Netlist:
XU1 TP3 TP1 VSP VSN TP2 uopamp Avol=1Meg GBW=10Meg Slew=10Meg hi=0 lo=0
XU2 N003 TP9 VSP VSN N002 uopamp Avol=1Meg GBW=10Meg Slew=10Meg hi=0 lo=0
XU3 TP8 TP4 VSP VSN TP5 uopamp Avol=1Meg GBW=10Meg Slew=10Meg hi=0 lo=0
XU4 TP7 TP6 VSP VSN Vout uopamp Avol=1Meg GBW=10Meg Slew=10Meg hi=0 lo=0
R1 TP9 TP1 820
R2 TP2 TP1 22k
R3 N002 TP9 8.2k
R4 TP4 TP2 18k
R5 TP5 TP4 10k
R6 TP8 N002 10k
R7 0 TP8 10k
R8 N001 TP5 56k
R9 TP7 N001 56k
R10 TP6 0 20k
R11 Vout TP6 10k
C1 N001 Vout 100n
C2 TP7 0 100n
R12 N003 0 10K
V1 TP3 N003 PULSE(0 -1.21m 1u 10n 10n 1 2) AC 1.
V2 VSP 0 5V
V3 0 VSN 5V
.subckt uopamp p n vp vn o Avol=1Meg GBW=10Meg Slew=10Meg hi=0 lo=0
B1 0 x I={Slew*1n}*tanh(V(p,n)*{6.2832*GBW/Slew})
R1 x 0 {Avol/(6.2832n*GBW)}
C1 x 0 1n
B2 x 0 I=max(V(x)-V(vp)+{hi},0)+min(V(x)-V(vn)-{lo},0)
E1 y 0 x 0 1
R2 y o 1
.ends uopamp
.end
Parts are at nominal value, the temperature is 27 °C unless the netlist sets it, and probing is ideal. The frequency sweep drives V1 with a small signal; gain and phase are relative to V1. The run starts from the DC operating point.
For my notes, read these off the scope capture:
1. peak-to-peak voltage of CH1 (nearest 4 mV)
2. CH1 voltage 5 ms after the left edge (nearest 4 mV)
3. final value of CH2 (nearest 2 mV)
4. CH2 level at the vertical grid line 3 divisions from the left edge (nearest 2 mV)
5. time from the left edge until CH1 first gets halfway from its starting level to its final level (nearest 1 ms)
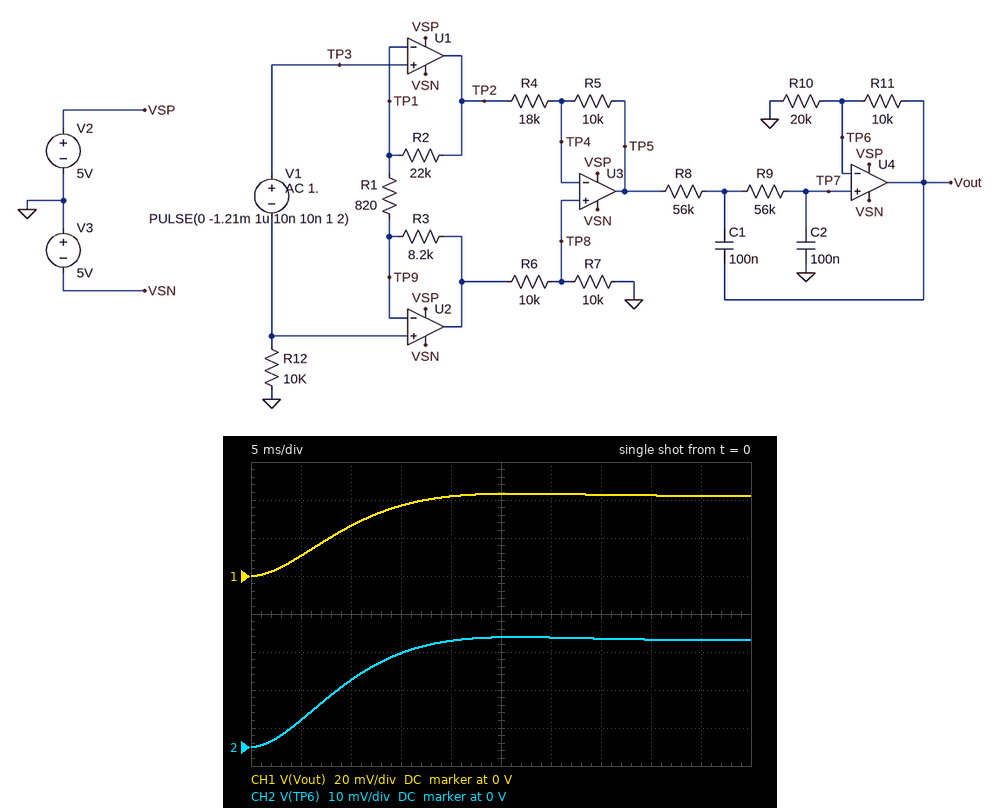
44 mV
12 mV
28 mV
24 mV
8 ms
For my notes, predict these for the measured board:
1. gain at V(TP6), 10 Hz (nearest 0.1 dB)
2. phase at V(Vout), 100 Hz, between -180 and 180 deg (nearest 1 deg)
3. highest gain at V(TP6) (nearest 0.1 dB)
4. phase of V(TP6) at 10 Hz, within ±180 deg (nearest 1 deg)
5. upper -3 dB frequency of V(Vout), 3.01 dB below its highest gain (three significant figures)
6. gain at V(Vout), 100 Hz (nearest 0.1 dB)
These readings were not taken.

27.1 dB
25 deg
27.3 dB
149 deg
26.7 Hz
8.9 dB
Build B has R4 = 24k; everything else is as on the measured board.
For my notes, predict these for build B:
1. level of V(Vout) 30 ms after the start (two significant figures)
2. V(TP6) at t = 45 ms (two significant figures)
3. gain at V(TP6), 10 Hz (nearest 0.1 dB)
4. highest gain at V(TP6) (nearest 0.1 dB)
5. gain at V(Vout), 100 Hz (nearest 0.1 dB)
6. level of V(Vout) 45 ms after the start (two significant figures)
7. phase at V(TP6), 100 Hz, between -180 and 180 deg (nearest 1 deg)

35 mV
23 mV
25.2 dB
25.4 dB
7.0 dB
34 mV
25 deg
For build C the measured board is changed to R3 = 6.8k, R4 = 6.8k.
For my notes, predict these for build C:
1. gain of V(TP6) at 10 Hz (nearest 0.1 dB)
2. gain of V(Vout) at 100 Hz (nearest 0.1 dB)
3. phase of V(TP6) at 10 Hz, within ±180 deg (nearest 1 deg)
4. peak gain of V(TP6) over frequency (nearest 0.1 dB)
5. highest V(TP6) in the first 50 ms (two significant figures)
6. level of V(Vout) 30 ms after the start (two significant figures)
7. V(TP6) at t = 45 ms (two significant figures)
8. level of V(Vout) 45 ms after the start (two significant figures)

34.0 dB
15.7 dB
149 deg
34.2 dB
64 mV
95 mV
62 mV
93 mV
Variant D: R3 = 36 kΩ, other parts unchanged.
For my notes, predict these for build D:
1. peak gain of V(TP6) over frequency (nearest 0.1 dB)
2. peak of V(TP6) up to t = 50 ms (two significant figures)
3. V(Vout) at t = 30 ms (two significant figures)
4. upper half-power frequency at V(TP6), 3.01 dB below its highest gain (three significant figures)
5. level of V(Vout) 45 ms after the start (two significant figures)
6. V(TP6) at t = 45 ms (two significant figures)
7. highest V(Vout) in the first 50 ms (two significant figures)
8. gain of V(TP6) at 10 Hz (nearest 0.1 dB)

33.9 dB
62 mV
92 mV
26.7 Hz
90 mV
60 mV
93 mV
33.7 dB
